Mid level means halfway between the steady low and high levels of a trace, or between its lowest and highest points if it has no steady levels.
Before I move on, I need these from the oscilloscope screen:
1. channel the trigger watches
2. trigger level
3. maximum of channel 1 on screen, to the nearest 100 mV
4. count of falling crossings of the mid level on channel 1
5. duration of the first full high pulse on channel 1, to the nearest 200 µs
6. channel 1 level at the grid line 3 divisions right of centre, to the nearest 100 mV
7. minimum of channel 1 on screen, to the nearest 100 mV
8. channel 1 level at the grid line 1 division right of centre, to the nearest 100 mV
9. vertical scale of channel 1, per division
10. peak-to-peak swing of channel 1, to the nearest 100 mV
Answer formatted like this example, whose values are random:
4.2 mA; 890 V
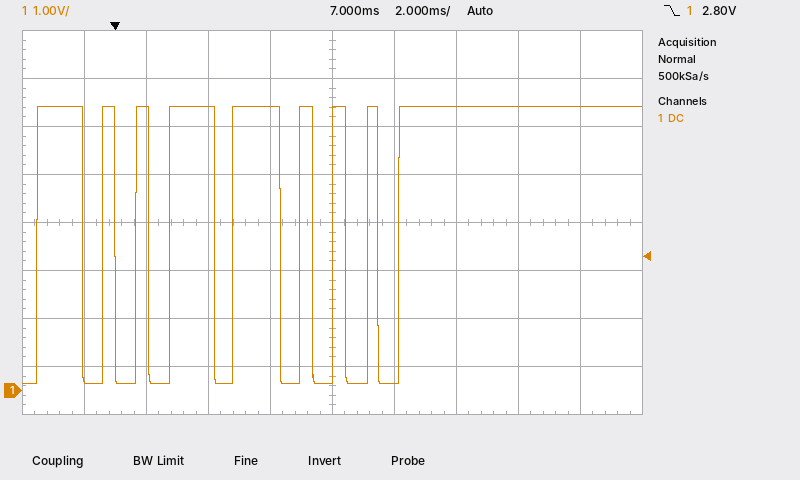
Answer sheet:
channel 1; 2.80 V; 5.9 V; 8; 1.4 ms; 5.9 V; 100 mV; 100 mV; 1 V; 5.8 V
